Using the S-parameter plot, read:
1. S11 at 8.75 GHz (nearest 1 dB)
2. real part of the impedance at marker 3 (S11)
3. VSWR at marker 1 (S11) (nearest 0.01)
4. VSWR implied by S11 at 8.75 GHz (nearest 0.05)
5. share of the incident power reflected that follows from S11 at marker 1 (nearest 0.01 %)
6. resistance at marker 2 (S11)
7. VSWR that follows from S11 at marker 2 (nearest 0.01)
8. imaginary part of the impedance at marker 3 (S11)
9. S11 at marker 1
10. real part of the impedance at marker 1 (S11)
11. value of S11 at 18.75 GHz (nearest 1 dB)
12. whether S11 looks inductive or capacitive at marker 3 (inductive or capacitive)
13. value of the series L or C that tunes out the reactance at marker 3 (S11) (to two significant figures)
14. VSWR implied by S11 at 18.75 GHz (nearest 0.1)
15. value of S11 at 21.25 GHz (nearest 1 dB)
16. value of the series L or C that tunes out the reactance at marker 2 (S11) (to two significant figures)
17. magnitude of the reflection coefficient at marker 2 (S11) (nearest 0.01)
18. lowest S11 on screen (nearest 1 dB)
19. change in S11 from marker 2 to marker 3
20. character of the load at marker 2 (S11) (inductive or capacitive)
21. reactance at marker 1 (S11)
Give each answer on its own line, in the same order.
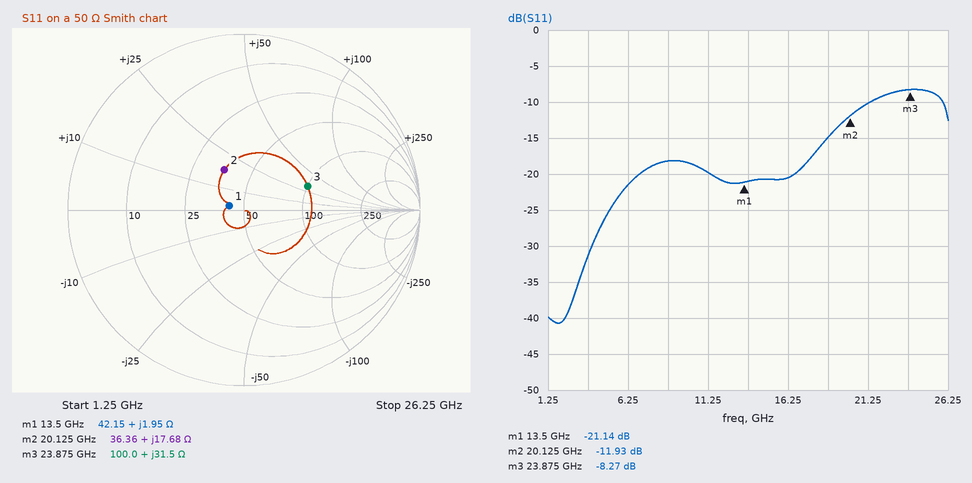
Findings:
-18 dB
100.0 Ω
1.19
1.30
0.77 %
36.36 Ω
1.68
+31.5 Ω
-21.14 dB
42.15 Ω
-15 dB
inductive
210 fF
1.4
-10 dB
450 fF
0.25
-41 dB
3.66 dB
inductive
+1.95 Ω
